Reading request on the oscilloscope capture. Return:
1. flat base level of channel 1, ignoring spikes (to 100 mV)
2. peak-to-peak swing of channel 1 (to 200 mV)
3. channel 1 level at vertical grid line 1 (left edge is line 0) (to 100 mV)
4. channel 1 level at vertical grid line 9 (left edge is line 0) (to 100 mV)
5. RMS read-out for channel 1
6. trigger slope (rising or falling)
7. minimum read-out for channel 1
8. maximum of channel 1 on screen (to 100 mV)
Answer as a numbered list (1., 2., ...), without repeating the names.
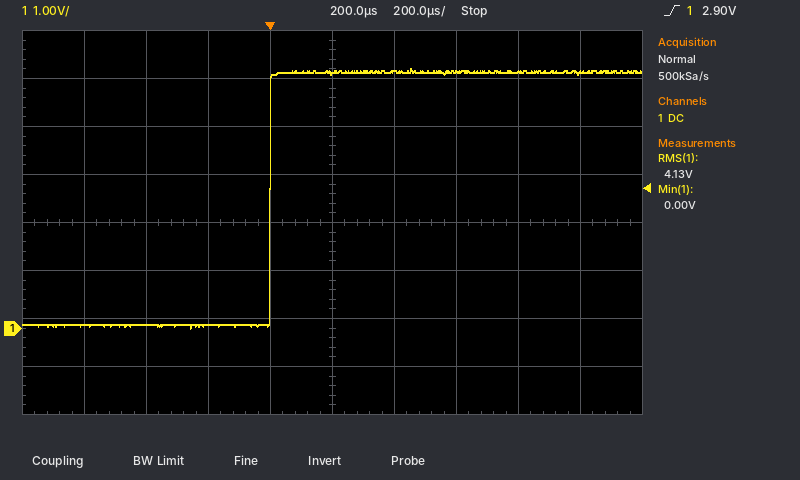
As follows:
1. 100 mV
2. 5.4 V
3. 100 mV
4. 5.3 V
5. 4.13 V
6. rising
7. 0.00 V
8. 5.4 V
